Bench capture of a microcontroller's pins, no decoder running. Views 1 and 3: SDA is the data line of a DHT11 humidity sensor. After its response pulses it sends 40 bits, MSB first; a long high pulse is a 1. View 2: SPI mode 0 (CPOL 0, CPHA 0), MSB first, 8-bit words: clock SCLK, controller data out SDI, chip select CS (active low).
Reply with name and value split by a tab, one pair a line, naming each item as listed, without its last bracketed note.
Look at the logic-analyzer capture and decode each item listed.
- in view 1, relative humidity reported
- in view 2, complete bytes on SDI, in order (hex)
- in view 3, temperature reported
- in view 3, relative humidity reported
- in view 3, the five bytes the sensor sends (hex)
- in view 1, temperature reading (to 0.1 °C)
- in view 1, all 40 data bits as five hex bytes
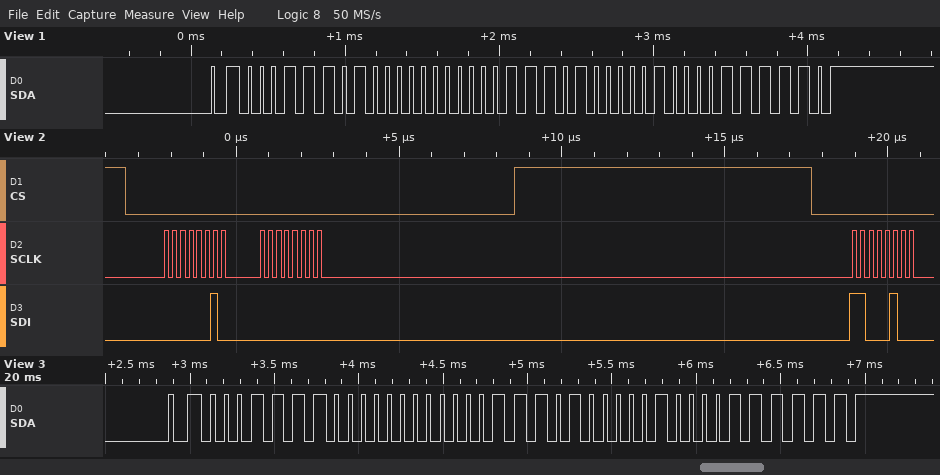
in view 1, relative humidity reported	29 %
in view 2, complete bytes on SDI, in order	0x02 0x00 0xC4
in view 3, temperature reported	29.4 °C
in view 3, relative humidity reported	30 %
in view 3, the five bytes the sensor sends	1E 00 1D 04 3F
in view 1, temperature reading	29.4 °C
in view 1, all 40 data bits as five hex bytes	1D 00 1D 04 3E
